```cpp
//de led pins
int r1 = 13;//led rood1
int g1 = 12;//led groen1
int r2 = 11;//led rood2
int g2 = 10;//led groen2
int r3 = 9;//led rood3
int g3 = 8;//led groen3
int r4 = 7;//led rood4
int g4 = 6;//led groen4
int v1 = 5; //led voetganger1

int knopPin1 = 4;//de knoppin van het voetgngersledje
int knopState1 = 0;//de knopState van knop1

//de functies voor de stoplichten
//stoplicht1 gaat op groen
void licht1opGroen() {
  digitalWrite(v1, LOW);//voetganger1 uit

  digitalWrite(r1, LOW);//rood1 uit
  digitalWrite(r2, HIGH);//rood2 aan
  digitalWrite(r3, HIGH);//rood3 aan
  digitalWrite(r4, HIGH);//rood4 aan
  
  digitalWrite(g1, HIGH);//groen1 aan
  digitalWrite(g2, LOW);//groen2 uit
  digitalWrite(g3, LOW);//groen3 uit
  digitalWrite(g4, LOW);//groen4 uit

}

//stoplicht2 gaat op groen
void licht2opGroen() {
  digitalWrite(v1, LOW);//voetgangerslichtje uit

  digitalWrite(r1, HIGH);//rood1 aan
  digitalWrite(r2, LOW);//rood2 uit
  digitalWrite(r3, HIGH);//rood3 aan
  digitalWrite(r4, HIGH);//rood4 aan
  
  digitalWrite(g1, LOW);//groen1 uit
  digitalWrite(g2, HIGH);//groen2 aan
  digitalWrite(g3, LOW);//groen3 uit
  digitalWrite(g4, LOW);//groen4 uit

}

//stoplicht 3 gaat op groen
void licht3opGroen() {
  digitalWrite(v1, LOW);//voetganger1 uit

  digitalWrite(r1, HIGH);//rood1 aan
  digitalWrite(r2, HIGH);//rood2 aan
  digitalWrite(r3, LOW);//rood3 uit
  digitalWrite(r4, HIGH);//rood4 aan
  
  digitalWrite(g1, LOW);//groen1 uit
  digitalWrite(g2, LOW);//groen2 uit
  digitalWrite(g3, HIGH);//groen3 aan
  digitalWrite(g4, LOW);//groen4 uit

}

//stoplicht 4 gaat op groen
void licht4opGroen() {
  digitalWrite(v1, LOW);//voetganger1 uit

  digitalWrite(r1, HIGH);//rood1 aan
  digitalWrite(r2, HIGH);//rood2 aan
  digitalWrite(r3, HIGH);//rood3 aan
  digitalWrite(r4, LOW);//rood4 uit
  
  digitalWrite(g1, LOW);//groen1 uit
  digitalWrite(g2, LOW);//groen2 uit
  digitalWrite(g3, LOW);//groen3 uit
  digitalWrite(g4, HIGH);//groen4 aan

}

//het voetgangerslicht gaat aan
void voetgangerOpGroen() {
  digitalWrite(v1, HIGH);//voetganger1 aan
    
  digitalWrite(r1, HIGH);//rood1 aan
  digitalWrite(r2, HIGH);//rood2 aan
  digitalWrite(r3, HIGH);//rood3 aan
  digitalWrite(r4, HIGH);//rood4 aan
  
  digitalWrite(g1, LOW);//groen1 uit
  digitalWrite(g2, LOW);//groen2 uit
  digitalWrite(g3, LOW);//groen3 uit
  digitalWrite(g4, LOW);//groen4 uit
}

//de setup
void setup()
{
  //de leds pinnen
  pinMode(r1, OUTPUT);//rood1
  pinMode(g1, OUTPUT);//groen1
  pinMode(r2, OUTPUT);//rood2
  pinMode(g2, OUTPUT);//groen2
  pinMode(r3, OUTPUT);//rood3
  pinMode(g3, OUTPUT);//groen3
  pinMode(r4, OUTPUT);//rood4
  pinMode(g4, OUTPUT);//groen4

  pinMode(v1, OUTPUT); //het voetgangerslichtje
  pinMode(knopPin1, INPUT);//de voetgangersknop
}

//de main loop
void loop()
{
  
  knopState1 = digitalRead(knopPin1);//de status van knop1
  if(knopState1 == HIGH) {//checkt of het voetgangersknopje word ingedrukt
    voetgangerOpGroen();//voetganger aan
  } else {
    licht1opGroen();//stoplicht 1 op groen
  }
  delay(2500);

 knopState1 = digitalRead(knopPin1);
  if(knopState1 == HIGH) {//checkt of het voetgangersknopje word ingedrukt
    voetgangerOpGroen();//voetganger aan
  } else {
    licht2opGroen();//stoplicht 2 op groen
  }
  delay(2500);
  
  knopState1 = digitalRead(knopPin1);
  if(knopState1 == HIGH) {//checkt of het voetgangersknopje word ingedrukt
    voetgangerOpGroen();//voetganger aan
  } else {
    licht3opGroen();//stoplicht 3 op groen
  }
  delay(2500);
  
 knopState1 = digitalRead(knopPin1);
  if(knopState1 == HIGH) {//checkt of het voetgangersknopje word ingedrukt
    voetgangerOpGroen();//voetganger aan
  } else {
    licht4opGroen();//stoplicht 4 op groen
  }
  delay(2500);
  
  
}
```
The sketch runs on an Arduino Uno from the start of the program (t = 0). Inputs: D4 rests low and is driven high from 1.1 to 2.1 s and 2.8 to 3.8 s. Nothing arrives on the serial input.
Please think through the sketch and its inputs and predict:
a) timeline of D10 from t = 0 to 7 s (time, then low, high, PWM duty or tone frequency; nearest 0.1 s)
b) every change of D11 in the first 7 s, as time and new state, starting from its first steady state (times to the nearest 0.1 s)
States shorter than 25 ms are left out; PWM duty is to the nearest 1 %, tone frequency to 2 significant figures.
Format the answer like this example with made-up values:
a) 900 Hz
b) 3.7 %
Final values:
a) 0 s low; 2.5 s high; 5 s low
b) 0 s high; 2.5 s low; 5 s high
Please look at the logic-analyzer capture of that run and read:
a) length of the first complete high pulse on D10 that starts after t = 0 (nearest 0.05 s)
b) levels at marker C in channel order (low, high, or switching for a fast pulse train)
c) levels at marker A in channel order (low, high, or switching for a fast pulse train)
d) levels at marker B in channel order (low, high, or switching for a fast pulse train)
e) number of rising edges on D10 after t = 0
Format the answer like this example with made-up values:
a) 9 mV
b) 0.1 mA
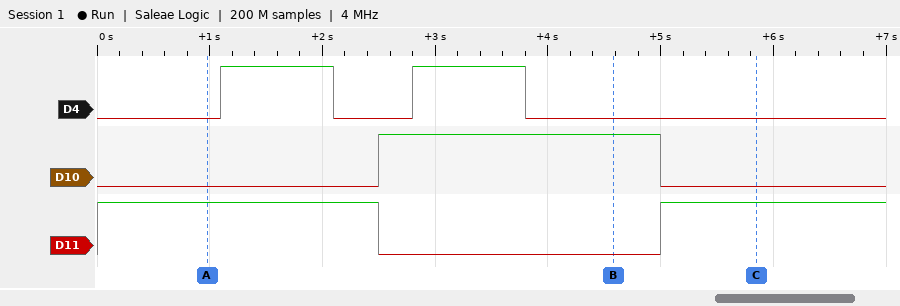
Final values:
a) 2.50 s
b) D4 low, D10 low, D11 high
c) D4 low, D10 low, D11 high
d) D4 low, D10 high, D11 low
e) 1
